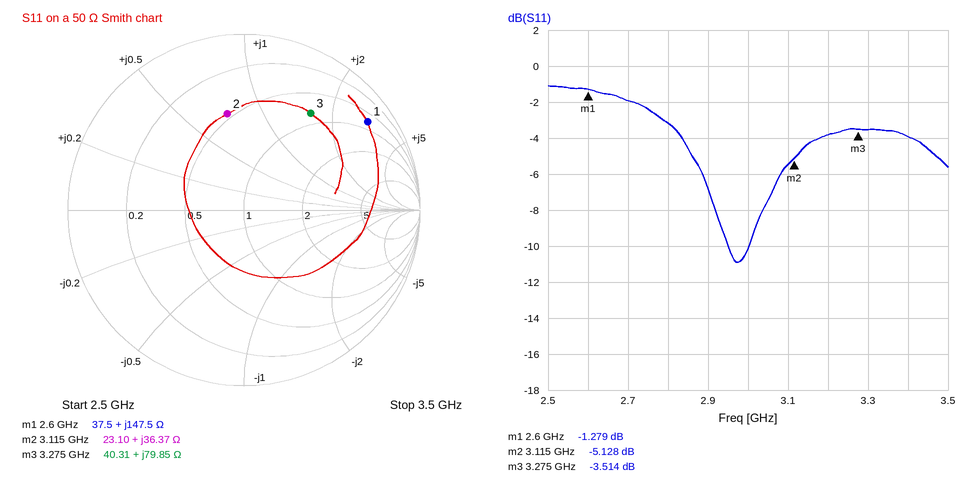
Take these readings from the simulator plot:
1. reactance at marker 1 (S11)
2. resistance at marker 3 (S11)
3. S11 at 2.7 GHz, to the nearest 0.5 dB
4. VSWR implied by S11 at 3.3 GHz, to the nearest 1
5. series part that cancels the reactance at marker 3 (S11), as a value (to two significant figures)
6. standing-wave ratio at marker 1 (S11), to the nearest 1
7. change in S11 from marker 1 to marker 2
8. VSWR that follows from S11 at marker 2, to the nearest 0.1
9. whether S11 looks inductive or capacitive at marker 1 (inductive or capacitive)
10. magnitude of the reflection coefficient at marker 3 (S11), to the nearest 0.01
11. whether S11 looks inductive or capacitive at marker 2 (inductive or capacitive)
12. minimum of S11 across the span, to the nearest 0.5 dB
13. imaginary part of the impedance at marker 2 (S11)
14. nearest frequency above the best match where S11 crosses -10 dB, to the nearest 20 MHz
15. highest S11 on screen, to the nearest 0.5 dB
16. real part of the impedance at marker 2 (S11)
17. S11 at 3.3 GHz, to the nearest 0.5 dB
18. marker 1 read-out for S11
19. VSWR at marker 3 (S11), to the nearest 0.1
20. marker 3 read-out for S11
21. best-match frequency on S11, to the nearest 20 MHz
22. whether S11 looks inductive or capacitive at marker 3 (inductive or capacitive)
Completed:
+147.5 Ω
40.31 Ω
-2.0 dB
5
610 fF
14
-3.849 dB
3.5
inductive
0.67
inductive
-11.0 dB
+36.37 Ω
3.00 GHz
-1.0 dB
23.10 Ω
-3.5 dB
-1.279 dB
5.0
-3.514 dB
2.98 GHz
inductive
